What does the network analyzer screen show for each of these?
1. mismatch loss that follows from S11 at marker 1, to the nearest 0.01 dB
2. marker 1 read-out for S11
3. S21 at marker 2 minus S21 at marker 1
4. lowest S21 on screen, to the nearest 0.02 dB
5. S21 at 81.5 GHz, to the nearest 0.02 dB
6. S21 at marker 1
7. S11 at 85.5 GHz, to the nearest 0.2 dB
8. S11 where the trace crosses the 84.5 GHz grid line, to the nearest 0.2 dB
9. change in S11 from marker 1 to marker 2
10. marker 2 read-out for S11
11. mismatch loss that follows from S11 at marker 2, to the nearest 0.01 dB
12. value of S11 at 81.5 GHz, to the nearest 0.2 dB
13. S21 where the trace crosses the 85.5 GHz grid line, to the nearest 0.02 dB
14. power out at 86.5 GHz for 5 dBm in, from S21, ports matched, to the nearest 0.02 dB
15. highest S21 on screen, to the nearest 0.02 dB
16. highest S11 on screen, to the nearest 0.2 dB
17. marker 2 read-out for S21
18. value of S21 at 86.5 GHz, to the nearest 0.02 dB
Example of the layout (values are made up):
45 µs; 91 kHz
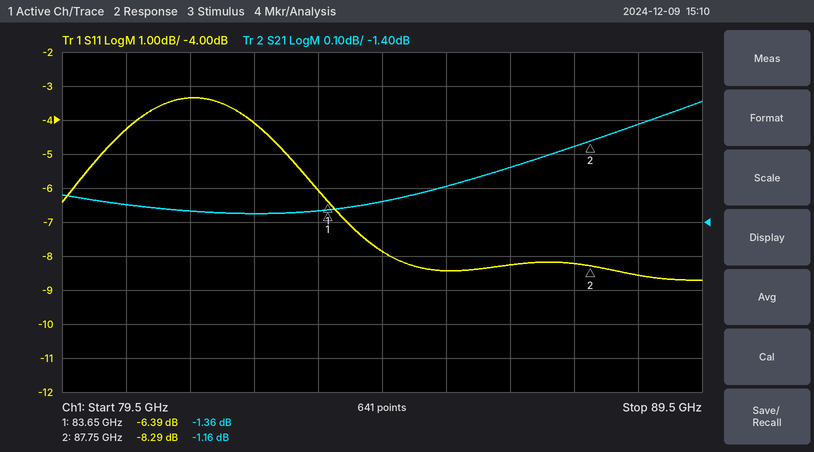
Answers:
1.13 dB; -6.39 dB; 0.20 dB; -1.38 dB; -1.36 dB; -1.36 dB; -8.4 dB; -7.8 dB; -1.90 dB; -8.29 dB; 0.70 dB; -3.4 dB; -1.30 dB; 3.76 dBm; -1.04 dB; -3.4 dB; -1.16 dB; -1.24 dB
